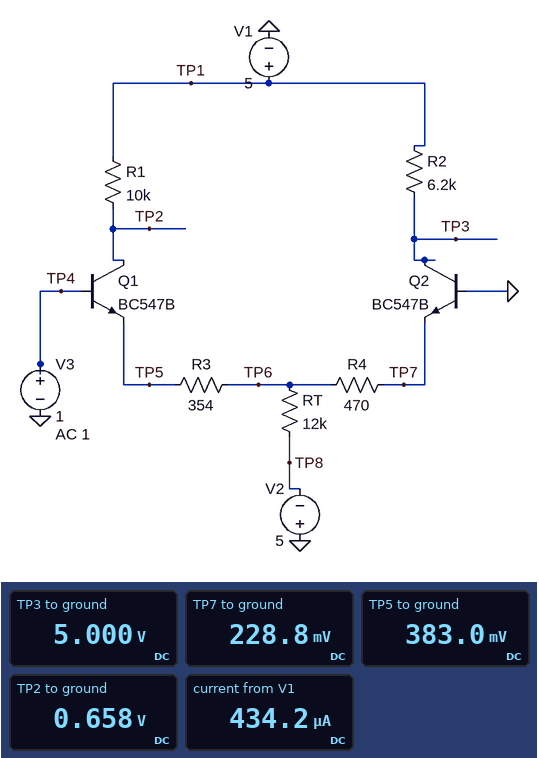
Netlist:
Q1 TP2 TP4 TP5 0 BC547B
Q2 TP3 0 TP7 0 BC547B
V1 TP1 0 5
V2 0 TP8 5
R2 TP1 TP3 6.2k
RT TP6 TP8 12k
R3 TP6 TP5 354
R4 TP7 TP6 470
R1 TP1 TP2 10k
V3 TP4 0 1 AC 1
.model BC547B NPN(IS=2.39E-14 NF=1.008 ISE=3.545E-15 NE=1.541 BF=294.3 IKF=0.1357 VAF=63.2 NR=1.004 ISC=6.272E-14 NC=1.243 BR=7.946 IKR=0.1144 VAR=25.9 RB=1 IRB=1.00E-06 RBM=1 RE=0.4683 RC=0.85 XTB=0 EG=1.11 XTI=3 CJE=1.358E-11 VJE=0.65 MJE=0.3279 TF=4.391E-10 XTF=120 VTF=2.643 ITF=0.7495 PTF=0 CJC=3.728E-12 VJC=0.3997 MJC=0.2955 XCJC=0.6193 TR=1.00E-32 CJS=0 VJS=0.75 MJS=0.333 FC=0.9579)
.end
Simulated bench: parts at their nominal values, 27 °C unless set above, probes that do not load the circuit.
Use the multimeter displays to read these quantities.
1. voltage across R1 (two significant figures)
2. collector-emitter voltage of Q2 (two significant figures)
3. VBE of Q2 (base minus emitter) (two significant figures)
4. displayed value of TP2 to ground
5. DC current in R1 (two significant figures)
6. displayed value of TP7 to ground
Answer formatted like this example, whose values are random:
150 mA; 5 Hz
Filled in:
4.3 V; 4.8 V; -230 mV; 0.658 V; 430 µA; 228.8 mV
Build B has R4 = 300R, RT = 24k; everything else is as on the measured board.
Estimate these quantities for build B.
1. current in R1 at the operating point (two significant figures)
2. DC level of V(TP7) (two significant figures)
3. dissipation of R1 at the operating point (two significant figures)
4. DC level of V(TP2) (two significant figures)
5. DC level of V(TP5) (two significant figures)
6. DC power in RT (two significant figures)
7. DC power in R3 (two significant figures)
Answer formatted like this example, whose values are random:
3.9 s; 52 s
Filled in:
220 µA; 320 mV; 490 µW; 2.8 V; 400 mV; 1.2 mW; 17 µW
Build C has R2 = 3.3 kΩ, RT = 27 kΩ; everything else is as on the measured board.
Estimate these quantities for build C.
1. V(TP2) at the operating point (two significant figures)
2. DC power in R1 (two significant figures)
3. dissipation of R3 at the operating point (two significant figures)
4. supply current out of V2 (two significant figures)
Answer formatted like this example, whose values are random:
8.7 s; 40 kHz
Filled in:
3.0 V; 390 µW; 14 µW; 200 µA
